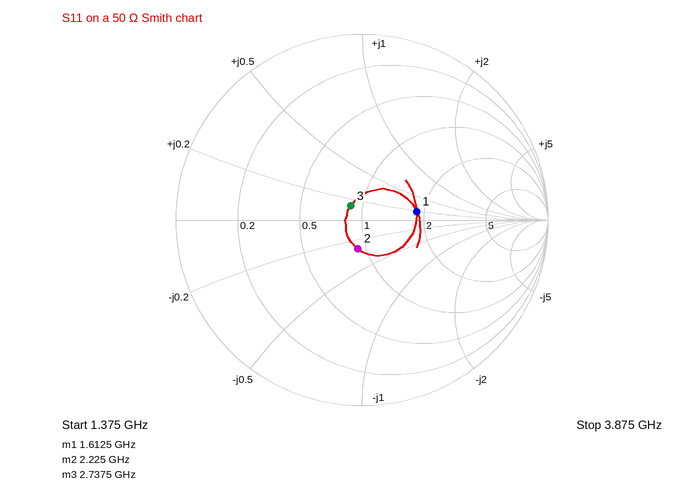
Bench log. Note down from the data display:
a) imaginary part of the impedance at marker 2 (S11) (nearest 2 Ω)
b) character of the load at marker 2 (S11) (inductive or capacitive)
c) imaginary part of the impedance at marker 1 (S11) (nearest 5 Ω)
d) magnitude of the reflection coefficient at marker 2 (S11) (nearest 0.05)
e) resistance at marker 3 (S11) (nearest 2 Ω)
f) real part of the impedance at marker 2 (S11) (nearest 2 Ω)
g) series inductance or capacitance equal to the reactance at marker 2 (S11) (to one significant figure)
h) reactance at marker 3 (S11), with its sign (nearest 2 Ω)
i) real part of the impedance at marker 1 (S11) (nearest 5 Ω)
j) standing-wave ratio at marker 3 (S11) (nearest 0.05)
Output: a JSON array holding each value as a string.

["-14 Ω", "capacitive", "+10 Ω", "0.15", "44 Ω", "46 Ω", "5 pF", "+6 Ω", "90 Ω", "1.20"]
